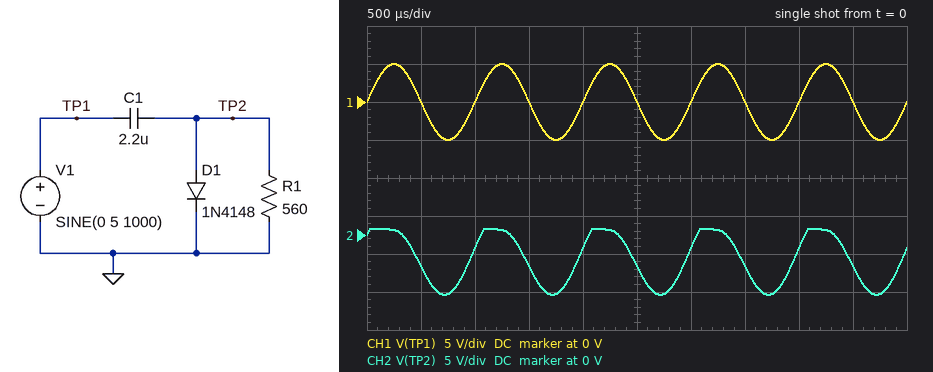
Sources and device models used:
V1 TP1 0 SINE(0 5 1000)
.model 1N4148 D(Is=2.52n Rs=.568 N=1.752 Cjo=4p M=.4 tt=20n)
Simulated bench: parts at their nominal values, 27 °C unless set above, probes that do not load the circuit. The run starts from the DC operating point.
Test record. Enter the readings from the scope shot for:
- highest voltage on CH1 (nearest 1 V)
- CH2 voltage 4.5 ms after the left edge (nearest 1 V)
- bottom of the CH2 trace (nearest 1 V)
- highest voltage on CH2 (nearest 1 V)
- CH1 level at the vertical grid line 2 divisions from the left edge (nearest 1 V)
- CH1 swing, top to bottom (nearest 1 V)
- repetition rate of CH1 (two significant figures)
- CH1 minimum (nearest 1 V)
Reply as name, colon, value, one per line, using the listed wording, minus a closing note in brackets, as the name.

highest voltage on CH1: 5 V
CH2 voltage 4.5 ms after the left edge: -4 V
bottom of the CH2 trace: -8 V
highest voltage on CH2: 1 V
CH1 level at the vertical grid line 2 divisions from the left edge: 0 V
CH1 swing, top to bottom: 10 V
repetition rate of CH1: 1.0 kHz
CH1 minimum: -5 V
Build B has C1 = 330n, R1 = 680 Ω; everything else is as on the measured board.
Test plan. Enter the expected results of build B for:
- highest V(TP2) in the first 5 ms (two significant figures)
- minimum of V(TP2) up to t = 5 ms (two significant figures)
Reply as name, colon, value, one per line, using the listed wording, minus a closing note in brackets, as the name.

highest V(TP2) in the first 5 ms: 690 mV
minimum of V(TP2) up to t = 5 ms: -4.6 V
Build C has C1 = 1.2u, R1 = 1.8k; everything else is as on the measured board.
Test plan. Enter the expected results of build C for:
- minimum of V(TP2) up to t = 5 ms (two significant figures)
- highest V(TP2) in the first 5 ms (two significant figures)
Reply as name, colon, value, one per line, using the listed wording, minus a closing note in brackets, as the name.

minimum of V(TP2) up to t = 5 ms: -8.5 V
highest V(TP2) in the first 5 ms: 770 mV
